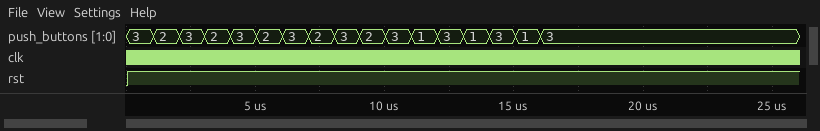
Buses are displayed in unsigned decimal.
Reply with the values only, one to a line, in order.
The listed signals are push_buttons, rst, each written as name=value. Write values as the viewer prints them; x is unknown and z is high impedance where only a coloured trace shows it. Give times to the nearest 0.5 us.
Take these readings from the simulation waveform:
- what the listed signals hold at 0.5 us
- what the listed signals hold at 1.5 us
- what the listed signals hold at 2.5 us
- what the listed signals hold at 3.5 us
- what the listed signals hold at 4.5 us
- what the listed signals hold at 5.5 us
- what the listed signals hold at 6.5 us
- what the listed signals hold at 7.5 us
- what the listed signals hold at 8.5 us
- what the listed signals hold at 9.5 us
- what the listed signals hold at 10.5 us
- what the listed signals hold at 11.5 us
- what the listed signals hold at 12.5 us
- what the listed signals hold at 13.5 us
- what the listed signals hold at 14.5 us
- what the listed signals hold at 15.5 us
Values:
push_buttons=3, rst=1
push_buttons=2, rst=1
push_buttons=3, rst=1
push_buttons=2, rst=1
push_buttons=3, rst=1
push_buttons=2, rst=1
push_buttons=3, rst=1
push_buttons=2, rst=1
push_buttons=3, rst=1
push_buttons=2, rst=1
push_buttons=3, rst=1
push_buttons=1, rst=1
push_buttons=3, rst=1
push_buttons=1, rst=1
push_buttons=3, rst=1
push_buttons=1, rst=1
